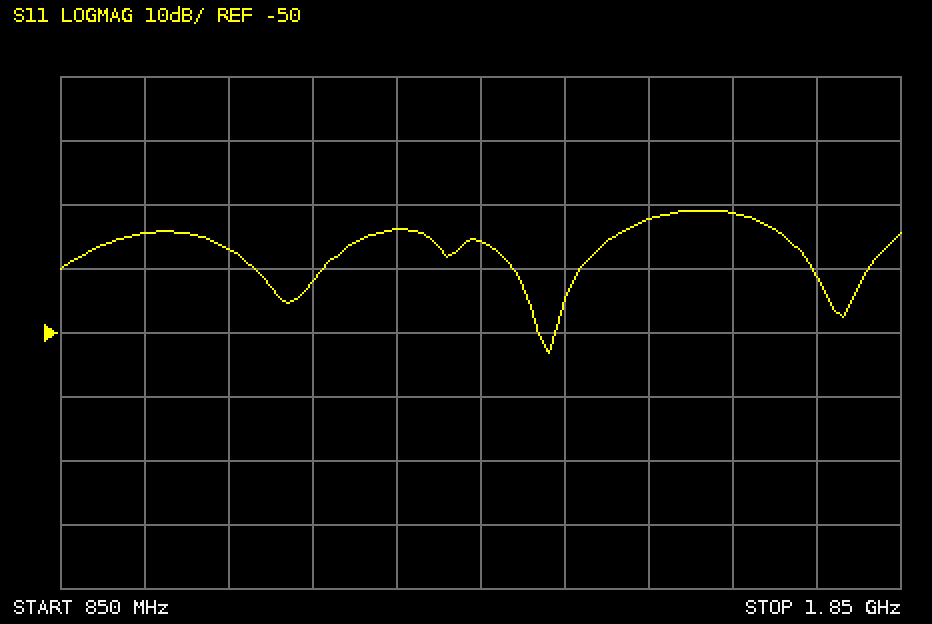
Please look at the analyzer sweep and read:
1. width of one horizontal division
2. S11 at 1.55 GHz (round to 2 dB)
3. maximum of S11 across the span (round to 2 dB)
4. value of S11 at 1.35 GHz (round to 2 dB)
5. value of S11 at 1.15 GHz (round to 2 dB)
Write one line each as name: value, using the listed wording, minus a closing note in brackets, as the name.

width of one horizontal division: 100 MHz
S11 at 1.55 GHz: -32 dB
maximum of S11 across the span: -30 dB
value of S11 at 1.35 GHz: -36 dB
value of S11 at 1.15 GHz: -42 dB
